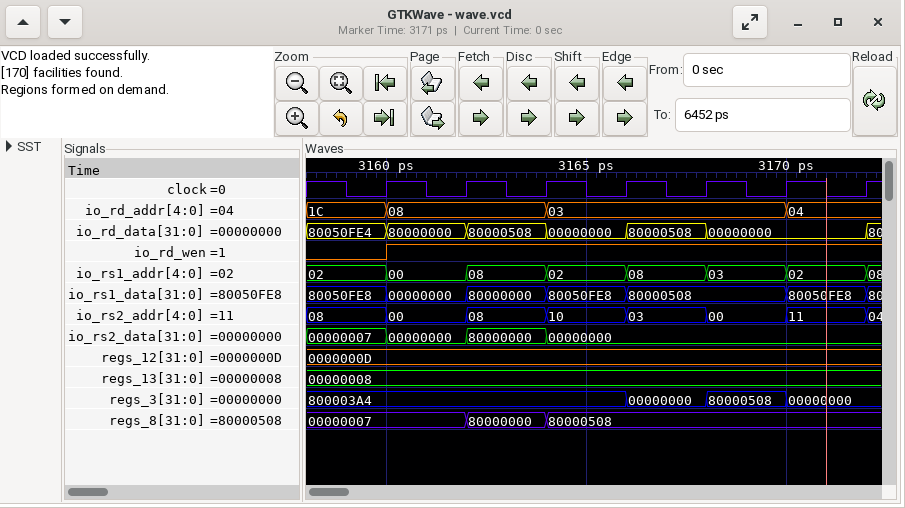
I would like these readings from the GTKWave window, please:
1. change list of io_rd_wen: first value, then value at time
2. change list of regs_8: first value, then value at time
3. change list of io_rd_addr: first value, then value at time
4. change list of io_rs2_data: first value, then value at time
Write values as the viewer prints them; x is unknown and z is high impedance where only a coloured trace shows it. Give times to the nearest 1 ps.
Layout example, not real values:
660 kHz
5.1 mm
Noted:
0, 1 at 3160 ps
00000007, 80000000 at 3162 ps, 80000508 at 3164 ps
1C, 08 at 3160 ps, 03 at 3164 ps, 04 at 3170 ps
00000007, 00000000 at 3160 ps, 80000000 at 3162 ps, 00000000 at 3164 ps
